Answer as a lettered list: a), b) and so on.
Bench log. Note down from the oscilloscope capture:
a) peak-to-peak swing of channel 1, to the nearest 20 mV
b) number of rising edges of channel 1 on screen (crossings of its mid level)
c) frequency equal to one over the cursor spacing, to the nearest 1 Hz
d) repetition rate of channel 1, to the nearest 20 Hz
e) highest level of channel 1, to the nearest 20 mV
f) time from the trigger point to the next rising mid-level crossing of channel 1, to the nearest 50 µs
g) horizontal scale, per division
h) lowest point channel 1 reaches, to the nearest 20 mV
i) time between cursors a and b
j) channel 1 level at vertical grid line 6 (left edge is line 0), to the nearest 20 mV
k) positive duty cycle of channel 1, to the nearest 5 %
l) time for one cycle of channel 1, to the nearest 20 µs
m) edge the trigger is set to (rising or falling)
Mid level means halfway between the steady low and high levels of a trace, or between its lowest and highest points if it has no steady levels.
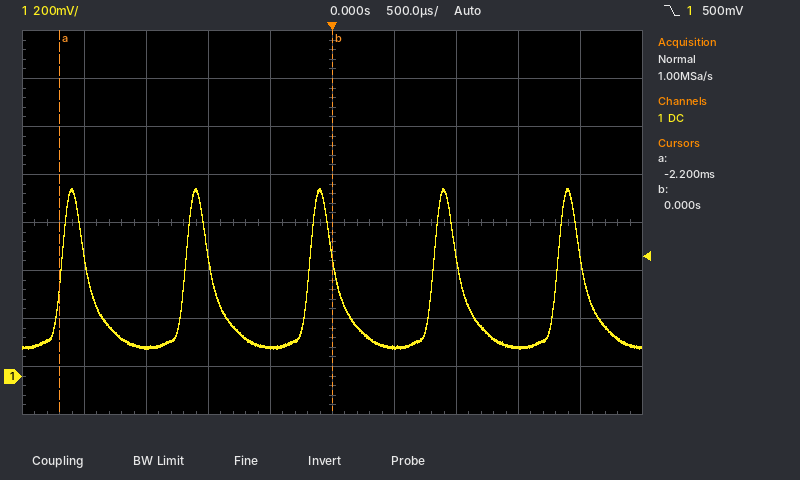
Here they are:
a) 660 mV
b) 5
c) 455 Hz
d) 1.00 kHz
e) 780 mV
f) 800 µs
g) 500 µs
h) 120 mV
i) 2.20 ms
j) 120 mV
k) 20 %
l) 1.00 ms
m) falling
